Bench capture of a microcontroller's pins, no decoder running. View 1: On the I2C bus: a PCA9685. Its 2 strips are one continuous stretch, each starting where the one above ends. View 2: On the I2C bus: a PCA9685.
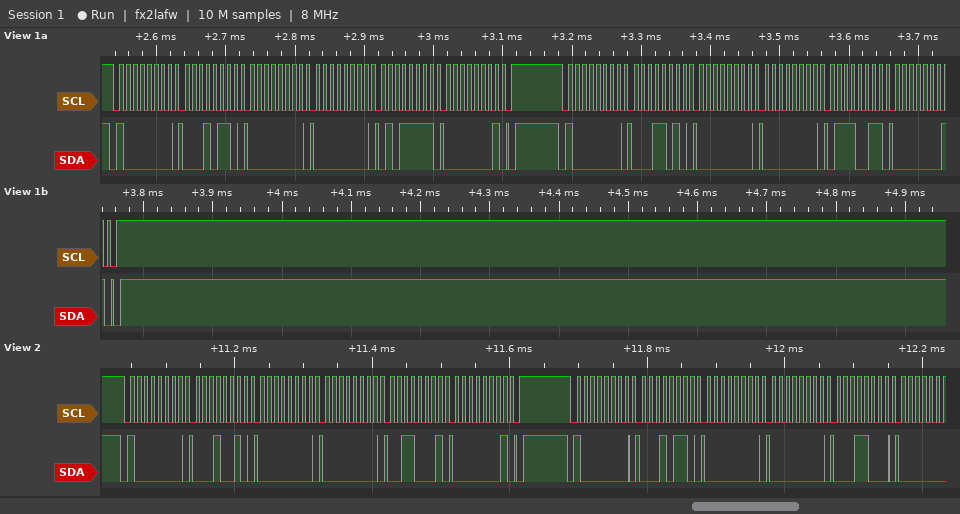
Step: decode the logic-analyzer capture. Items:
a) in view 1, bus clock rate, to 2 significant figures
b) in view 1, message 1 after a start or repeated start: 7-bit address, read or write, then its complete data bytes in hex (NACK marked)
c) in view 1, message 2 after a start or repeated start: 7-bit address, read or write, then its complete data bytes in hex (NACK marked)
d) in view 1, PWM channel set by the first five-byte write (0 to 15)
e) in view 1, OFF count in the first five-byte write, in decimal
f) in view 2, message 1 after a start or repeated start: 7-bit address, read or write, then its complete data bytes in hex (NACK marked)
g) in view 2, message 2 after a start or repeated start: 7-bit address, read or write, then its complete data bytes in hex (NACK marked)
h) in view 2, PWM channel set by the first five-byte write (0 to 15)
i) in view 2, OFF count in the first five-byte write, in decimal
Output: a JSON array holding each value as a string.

["100 kHz", "0x40 write: 16 00 00 5F 01", "0x40 write: 1A 00 00 73 01", "4", "351", "0x40 write: 12 00 00 31 01", "0x40 write: 16 00 00 18", "3", "305"]
